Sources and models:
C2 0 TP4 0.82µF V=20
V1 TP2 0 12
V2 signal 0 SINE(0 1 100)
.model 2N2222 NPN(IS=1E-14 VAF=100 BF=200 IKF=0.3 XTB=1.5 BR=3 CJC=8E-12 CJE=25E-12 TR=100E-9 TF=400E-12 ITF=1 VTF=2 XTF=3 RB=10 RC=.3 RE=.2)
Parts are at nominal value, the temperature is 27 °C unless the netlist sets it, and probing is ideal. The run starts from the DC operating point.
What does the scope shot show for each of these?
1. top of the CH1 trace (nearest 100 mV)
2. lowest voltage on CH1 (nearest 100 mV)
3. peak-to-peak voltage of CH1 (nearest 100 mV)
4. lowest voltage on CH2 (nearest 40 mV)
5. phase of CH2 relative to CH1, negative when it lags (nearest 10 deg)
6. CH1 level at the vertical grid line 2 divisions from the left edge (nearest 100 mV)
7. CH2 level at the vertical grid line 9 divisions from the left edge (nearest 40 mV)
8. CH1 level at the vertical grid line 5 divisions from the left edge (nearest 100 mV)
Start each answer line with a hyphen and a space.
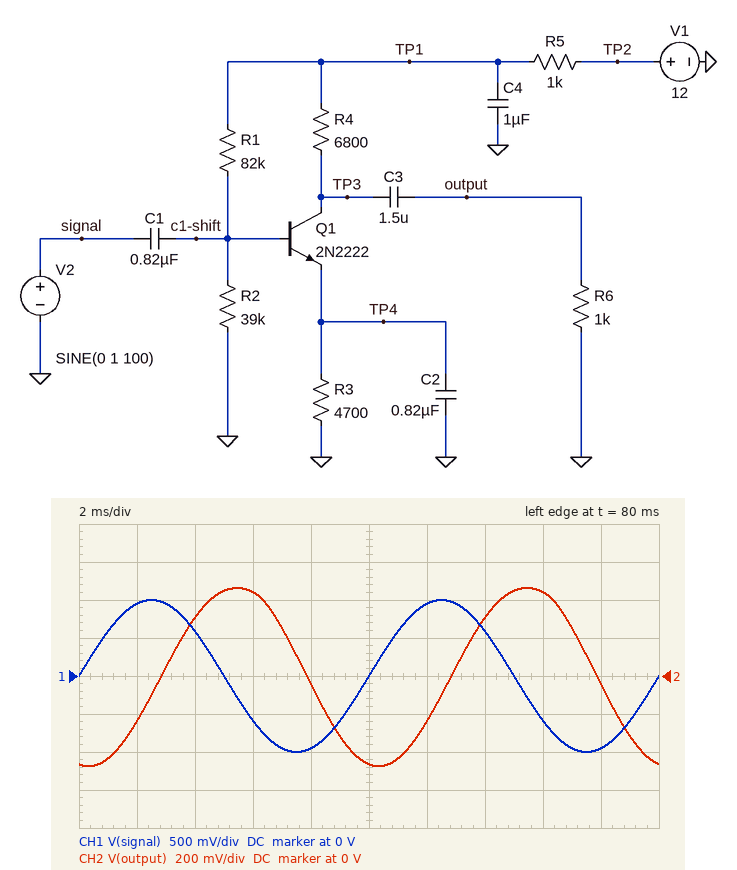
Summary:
- 1.0 V
- -1.0 V
- 2.0 V
- -480 mV
- -100 deg
- 600 mV
- -40 mV
- 0 V
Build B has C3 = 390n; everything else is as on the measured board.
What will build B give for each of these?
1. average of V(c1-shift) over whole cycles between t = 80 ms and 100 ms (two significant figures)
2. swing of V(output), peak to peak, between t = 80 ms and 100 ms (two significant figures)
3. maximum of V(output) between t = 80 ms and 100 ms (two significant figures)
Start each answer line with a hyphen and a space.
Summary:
- 3.6 V
- 840 mV
- 410 mV
